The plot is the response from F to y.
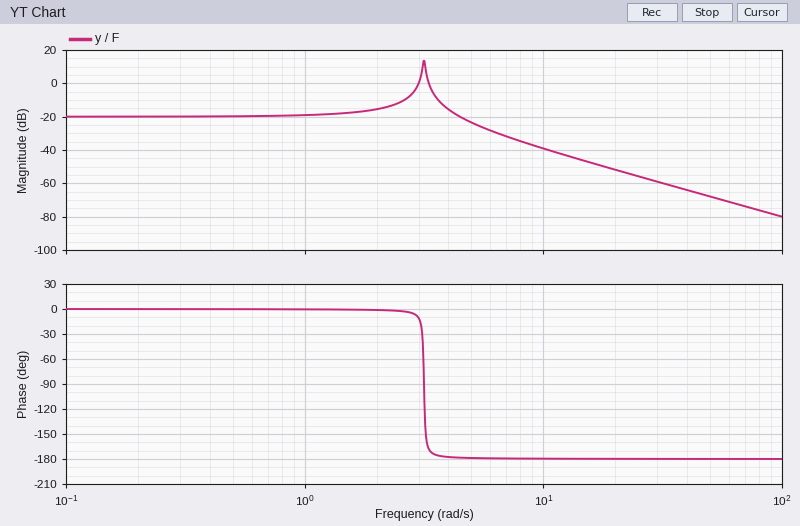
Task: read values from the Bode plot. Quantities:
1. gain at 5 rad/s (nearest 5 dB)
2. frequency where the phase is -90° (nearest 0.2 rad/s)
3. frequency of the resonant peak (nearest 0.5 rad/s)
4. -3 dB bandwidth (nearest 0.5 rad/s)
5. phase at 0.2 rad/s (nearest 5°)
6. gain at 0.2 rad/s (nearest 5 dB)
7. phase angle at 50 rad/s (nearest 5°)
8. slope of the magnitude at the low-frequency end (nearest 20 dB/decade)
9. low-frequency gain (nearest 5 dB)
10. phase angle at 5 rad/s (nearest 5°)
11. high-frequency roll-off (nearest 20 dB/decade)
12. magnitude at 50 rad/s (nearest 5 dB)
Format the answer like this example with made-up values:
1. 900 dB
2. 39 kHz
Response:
1. -25 dB
2. 3.2 rad/s
3. 3.0 rad/s
4. 5.0 rad/s
5. 0°
6. -20 dB
7. -180°
8. 0 dB/decade
9. -20 dB
10. -180°
11. -40 dB/decade
12. -70 dB
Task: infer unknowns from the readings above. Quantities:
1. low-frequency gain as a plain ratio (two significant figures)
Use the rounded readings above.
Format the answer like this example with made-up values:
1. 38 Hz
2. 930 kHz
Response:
1. 0.10
